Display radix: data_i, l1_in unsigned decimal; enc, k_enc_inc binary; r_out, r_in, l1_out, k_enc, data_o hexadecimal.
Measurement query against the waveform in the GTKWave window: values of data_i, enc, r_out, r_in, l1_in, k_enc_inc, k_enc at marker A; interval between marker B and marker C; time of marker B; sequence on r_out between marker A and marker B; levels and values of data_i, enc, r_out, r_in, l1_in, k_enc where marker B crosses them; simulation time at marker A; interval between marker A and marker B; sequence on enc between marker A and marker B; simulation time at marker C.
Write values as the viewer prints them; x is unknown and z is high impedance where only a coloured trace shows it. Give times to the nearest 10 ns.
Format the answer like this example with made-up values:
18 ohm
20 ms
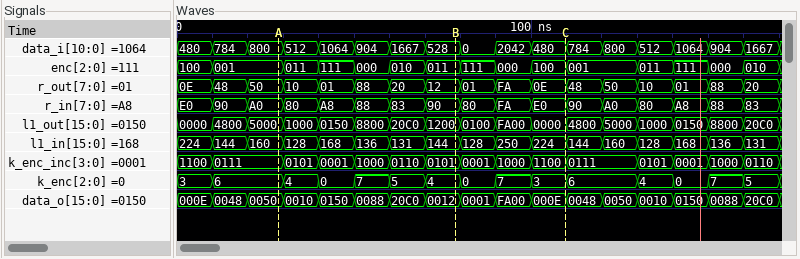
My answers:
data_i=800, enc=001, r_out=50, r_in=A0, l1_in=160, k_enc_inc=0111, k_enc=6
30 ns
80 ns
50, 10, 01, 88, 20, 12
data_i=528, enc=011, r_out=12, r_in=90, l1_in=144, k_enc=4
30 ns
50 ns
001, 011, 111, 000, 010, 011
110 ns
